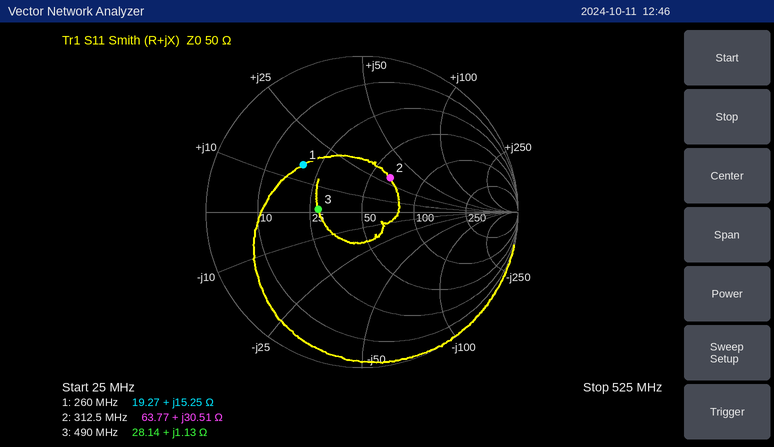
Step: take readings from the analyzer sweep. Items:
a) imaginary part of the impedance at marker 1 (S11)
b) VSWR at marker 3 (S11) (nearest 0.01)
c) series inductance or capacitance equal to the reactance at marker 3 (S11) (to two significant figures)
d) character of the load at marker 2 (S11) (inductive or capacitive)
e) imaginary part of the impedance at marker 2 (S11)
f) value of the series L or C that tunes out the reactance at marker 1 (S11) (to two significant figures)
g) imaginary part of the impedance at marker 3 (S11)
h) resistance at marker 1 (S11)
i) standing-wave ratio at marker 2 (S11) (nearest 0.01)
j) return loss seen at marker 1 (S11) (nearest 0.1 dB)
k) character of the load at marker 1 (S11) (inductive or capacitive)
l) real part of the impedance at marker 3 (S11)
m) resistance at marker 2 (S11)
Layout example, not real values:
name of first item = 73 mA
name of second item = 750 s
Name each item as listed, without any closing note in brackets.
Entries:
imaginary part of the impedance at marker 1 = +15.25 Ω
VSWR at marker 3 (S11) = 1.78
series inductance or capacitance equal to the reactance at marker 3 (S11) = 370 pH
character of the load at marker 2 (S11) = inductive
imaginary part of the impedance at marker 2 = +30.51 Ω
value of the series L or C that tunes out the reactance at marker 1 (S11) = 40 pF
imaginary part of the impedance at marker 3 = +1.13 Ω
resistance at marker 1 = 19.27 Ω
standing-wave ratio at marker 2 (S11) = 1.79
return loss seen at marker 1 (S11) = 6.3 dB
character of the load at marker 1 (S11) = inductive
real part of the impedance at marker 3 = 28.14 Ω
resistance at marker 2 = 63.77 Ω
